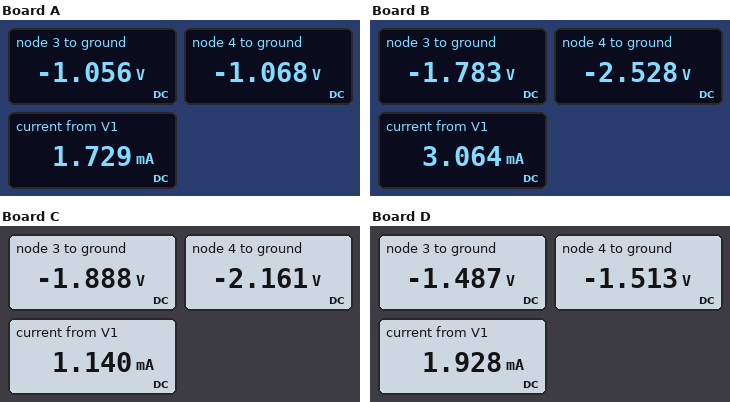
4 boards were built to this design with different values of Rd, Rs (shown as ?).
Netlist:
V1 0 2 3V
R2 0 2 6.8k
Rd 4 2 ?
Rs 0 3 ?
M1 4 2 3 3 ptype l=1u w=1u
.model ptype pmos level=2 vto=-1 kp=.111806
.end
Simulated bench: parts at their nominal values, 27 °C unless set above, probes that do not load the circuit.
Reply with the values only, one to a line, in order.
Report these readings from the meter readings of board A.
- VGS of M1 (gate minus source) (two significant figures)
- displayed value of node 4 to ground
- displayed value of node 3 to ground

-1.9 V
-1.068 V
-1.056 V
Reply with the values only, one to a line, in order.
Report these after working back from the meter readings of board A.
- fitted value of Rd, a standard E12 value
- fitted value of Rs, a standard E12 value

1.5 kΩ
820 Ω
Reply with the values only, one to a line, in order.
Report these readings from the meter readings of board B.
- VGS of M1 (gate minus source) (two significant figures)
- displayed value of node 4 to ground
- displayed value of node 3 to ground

-1.2 V
-2.528 V
-1.783 V
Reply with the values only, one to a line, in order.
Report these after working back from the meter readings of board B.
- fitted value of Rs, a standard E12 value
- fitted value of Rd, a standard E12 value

680 Ω
180 Ω
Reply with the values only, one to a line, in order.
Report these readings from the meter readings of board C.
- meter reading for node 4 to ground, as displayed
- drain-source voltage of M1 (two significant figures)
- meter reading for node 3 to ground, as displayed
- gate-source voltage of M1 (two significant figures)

-2.161 V
-270 mV
-1.888 V
-1.1 V
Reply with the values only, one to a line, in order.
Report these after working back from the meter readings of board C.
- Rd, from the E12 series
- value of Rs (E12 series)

1.2 kΩ
2.7 kΩ
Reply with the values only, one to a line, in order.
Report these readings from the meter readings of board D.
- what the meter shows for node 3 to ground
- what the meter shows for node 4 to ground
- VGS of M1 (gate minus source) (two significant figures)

-1.487 V
-1.513 V
-1.5 V
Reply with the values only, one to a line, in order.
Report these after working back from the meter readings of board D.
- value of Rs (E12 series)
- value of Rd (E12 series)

1 kΩ
1 kΩ
